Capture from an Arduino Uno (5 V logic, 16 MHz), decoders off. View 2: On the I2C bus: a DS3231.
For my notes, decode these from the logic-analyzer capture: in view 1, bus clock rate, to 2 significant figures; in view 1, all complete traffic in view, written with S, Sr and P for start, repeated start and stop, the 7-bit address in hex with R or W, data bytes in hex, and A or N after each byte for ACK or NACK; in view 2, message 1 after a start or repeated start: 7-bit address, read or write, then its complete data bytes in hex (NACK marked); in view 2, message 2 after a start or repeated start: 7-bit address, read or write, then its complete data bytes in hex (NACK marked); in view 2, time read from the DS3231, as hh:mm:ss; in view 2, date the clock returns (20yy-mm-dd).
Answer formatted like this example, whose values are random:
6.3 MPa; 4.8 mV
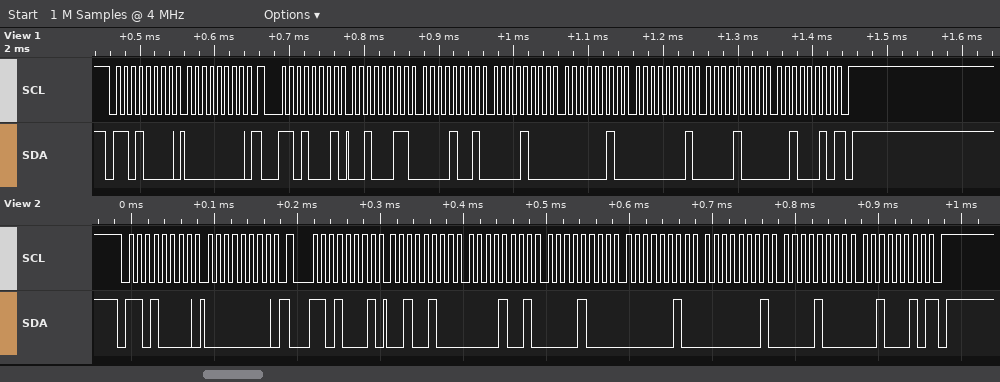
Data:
100 kHz; S 68W A 00 A Sr 68R A 23 A 09 A 08 A 02 A 01 A 08 A 22 N P; 0x68 write: 00; 0x68 read: 24 09 08 02 01 08 22 NACK; 08:09:24; 2022-08-01
